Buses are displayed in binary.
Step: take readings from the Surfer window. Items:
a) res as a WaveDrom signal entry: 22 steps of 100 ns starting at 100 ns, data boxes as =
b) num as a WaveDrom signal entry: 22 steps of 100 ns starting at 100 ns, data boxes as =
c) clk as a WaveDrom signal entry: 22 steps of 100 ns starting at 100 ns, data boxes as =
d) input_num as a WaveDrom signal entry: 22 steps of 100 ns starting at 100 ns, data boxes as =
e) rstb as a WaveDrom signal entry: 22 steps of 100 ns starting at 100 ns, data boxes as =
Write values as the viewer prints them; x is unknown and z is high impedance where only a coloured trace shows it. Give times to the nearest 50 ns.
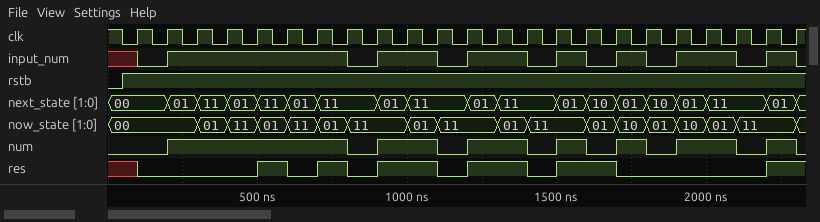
{name: 'res', wave: '0...10101.01.01.0....1'}
{name: 'num', wave: '01.....01.01.010101.01'}
{name: 'clk', wave: 'p.....................'}
{name: 'input_num', wave: '01.....01.01.010101.01'}
{name: 'rstb', wave: '1.....................'}
